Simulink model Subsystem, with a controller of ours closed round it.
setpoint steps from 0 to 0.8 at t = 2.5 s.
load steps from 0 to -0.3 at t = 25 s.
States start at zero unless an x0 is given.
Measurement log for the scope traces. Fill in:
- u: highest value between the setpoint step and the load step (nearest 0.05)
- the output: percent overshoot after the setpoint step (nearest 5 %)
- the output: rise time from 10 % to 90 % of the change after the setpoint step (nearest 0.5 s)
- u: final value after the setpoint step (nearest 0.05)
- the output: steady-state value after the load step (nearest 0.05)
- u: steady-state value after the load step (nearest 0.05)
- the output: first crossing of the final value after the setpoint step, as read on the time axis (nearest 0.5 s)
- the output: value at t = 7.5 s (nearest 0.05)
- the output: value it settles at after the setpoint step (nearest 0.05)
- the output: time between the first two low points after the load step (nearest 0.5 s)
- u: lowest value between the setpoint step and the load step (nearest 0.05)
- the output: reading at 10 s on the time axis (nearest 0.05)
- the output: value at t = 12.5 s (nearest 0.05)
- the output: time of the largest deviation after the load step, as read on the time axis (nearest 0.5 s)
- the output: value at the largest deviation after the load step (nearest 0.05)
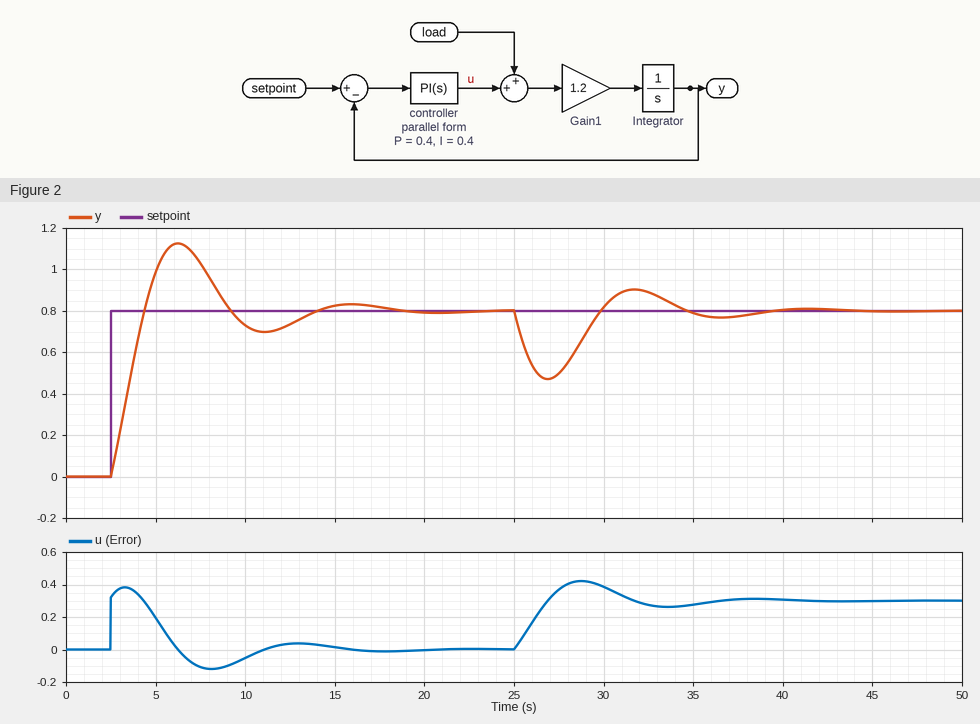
0.40
40 %
1.5 s
0.00
0.80
0.30
4.5 s
1.05
0.80
9.5 s
-0.10
0.75
0.75
27.0 s
0.45
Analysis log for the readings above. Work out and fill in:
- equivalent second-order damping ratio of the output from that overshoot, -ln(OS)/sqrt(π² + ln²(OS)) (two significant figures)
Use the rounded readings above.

0.28
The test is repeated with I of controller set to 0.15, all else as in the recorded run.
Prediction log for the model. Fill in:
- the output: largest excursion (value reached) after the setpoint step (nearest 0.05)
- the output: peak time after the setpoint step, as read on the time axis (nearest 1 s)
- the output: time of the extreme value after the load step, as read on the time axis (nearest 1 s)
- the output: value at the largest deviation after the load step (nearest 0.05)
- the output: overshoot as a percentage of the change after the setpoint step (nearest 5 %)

1.00
8 s
28 s
0.35
25 %
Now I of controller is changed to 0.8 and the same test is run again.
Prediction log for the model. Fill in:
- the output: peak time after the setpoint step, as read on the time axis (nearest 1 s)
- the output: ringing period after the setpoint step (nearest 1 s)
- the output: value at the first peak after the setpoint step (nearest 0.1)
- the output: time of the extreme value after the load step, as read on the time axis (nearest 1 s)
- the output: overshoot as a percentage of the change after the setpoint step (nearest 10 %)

5 s
7 s
1.2
26 s
50 %
